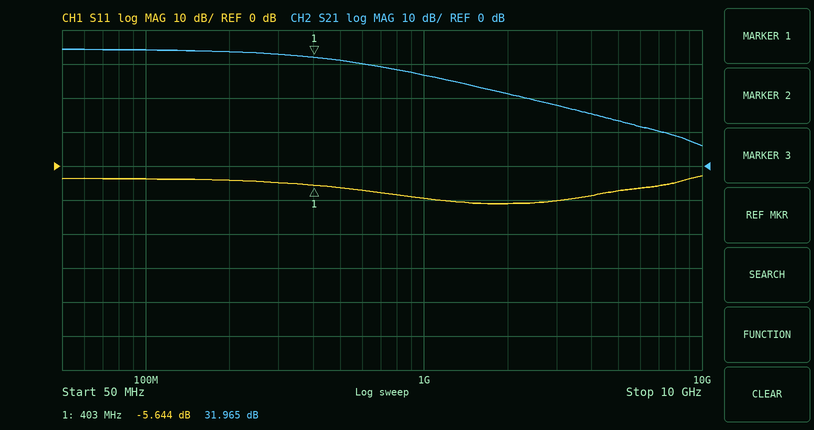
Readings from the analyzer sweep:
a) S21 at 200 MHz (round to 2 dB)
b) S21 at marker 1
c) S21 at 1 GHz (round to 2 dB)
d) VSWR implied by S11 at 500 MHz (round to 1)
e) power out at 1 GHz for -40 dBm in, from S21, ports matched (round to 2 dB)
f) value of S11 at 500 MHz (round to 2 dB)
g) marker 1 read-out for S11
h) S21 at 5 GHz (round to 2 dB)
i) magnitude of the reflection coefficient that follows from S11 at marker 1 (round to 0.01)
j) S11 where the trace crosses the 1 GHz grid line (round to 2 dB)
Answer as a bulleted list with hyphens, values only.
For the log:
- 34 dB
- 31.965 dB
- 26 dB
- 3
- -14 dBm
- -6 dB
- -5.644 dB
- 14 dB
- 0.52
- -10 dB
